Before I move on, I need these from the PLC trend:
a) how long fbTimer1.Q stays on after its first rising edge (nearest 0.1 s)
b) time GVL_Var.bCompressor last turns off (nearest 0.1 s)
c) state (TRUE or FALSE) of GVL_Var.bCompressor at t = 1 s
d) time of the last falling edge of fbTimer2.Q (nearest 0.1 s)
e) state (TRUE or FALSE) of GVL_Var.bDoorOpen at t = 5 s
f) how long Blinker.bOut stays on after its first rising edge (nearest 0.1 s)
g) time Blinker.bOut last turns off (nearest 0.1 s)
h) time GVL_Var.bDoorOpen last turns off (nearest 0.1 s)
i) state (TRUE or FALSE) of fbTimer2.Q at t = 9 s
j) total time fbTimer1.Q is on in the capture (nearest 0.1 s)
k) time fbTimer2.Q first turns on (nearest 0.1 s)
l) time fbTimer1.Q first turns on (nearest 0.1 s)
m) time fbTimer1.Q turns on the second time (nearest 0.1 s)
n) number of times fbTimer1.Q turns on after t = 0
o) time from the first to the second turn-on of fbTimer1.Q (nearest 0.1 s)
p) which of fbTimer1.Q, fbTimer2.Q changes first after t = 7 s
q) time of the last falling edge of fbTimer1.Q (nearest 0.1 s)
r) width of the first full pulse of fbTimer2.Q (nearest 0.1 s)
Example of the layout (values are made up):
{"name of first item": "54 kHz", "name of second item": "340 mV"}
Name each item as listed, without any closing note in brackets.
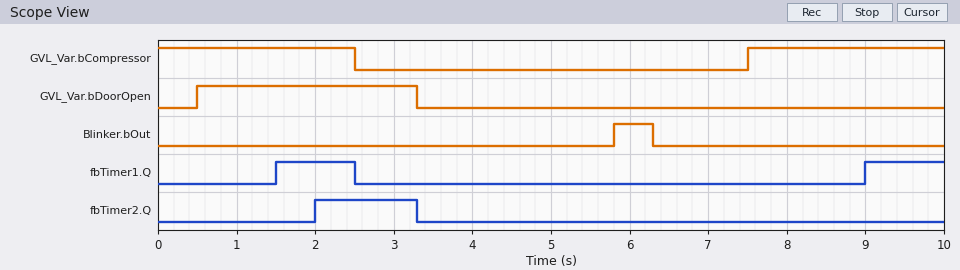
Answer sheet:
{"how long fbTimer1.Q stays on after its first rising edge": "1.0 s", "time GVL_Var.bCompressor last turns off": "2.5 s", "state (TRUE or FALSE) of GVL_Var.bCompressor at t = 1 s": "TRUE", "time of the last falling edge of fbTimer2.Q": "3.3 s", "state (TRUE or FALSE) of GVL_Var.bDoorOpen at t = 5 s": "FALSE", "how long Blinker.bOut stays on after its first rising edge": "0.5 s", "time Blinker.bOut last turns off": "6.3 s", "time GVL_Var.bDoorOpen last turns off": "3.3 s", "state (TRUE or FALSE) of fbTimer2.Q at t = 9 s": "FALSE", "total time fbTimer1.Q is on in the capture": "2.0 s", "time fbTimer2.Q first turns on": "2.0 s", "time fbTimer1.Q first turns on": "1.5 s", "time fbTimer1.Q turns on the second time": "9.0 s", "number of times fbTimer1.Q turns on after t = 0": "2", "time from the first to the second turn-on of fbTimer1.Q": "7.5 s", "which of fbTimer1.Q, fbTimer2.Q changes first after t = 7 s": "fbTimer1.Q", "time of the last falling edge of fbTimer1.Q": "2.5 s", "width of the first full pulse of fbTimer2.Q": "1.3 s"}
